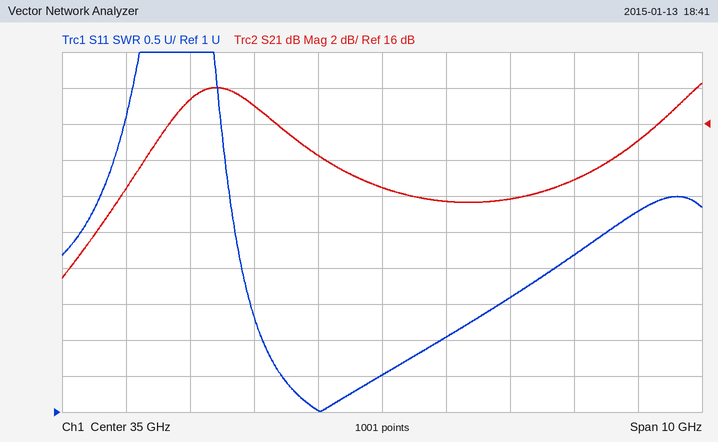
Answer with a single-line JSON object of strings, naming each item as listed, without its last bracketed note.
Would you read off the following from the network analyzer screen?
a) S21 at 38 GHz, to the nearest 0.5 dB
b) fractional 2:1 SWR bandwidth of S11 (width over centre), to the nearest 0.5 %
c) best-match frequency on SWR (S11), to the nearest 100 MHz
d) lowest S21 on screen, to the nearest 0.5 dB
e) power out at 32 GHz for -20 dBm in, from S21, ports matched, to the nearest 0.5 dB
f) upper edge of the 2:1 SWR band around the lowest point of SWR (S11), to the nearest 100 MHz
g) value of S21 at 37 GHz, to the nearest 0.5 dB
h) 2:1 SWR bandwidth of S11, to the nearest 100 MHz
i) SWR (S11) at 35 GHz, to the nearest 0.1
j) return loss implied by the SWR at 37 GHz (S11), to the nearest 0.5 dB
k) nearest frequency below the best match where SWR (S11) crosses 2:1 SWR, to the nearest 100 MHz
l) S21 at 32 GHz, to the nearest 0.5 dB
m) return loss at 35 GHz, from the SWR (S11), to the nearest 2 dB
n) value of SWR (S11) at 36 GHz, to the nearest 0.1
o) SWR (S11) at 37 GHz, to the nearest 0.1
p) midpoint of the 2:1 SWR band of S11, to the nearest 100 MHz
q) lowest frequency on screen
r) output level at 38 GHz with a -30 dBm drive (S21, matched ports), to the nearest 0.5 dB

{"S21 at 38 GHz, to the nearest 0.5 dB": "13.0 dB", "fractional 2:1 SWR bandwidth of S11 (width over centre), to the nearest 0.5 %": "8.0 %", "best-match frequency on SWR (S11), to the nearest 100 MHz": "34.0 GHz", "lowest S21 on screen, to the nearest 0.5 dB": "7.5 dB", "power out at 32 GHz for -20 dBm in, from S21, ports matched, to the nearest 0.5 dB": "-2.5 dBm", "upper edge of the 2:1 SWR band around the lowest point of SWR (S11), to the nearest 100 MHz": "35.9 GHz", "value of S21 at 37 GHz, to the nearest 0.5 dB": "12.0 dB", "2:1 SWR bandwidth of S11, to the nearest 100 MHz": "2.8 GHz", "SWR (S11) at 35 GHz, to the nearest 0.1": "1.5", "return loss implied by the SWR at 37 GHz (S11), to the nearest 0.5 dB": "7.0 dB", "nearest frequency below the best match where SWR (S11) crosses 2:1 SWR, to the nearest 100 MHz": "33.1 GHz", "S21 at 32 GHz, to the nearest 0.5 dB": "17.5 dB", "return loss at 35 GHz, from the SWR (S11), to the nearest 2 dB": "14 dB", "value of SWR (S11) at 36 GHz, to the nearest 0.1": "2.0", "SWR (S11) at 37 GHz, to the nearest 0.1": "2.6", "midpoint of the 2:1 SWR band of S11, to the nearest 100 MHz": "34.5 GHz", "lowest frequency on screen": "30 GHz", "output level at 38 GHz with a -30 dBm drive (S21, matched ports), to the nearest 0.5 dB": "-17.0 dBm"}
